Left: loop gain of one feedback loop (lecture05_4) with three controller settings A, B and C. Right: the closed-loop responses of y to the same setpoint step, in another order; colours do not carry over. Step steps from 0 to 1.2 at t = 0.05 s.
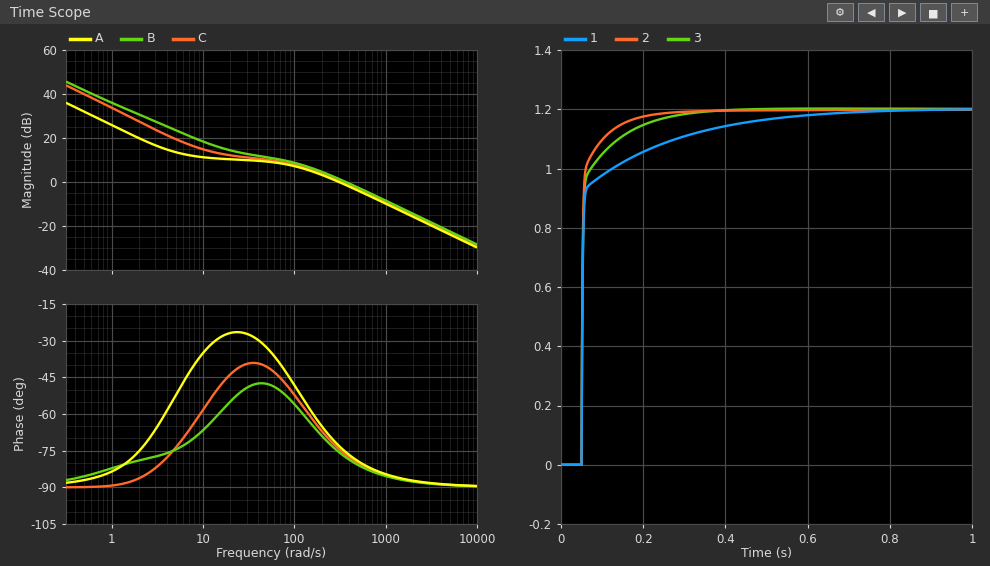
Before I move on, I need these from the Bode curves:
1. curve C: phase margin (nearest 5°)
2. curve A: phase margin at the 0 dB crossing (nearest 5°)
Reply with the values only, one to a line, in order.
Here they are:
105°
105°
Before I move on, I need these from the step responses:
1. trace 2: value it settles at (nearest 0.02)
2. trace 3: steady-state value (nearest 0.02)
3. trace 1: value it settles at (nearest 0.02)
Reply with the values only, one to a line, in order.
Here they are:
1.20
1.20
1.20
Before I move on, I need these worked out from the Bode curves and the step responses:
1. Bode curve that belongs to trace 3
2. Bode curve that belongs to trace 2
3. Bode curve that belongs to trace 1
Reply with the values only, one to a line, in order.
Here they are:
C
B
A
